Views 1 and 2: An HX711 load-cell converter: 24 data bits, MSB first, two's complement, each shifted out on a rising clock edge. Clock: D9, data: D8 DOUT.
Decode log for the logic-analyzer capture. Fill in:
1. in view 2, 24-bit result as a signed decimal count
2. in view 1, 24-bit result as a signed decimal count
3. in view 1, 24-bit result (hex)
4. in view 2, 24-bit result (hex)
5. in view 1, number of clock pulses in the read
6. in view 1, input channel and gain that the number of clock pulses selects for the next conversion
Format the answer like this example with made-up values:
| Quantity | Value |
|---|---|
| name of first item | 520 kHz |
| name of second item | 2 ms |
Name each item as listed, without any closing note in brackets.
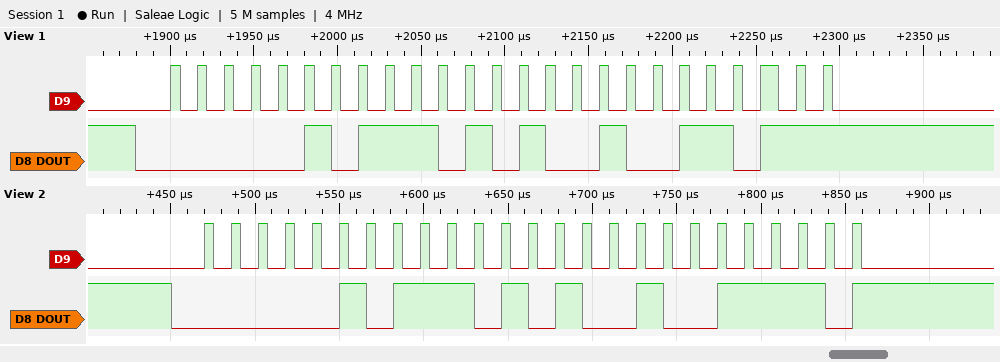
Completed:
| Quantity | Value |
|---|---|
| in view 2, 24-bit result as a signed decimal count | 382110 |
| in view 1, 24-bit result as a signed decimal count | 382107 |
| in view 1, 24-bit result | 0x05D49B |
| in view 2, 24-bit result | 0x05D49E |
| in view 1, number of clock pulses in the read | 25 |
| in view 1, input channel and gain that the number of clock pulses selects for the next conversion | channel A, gain 128 |
